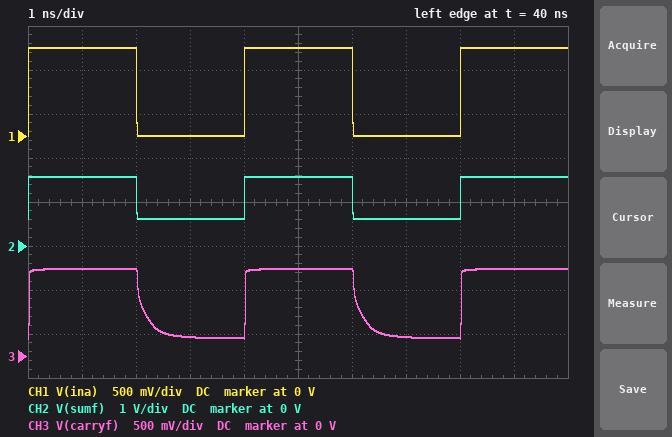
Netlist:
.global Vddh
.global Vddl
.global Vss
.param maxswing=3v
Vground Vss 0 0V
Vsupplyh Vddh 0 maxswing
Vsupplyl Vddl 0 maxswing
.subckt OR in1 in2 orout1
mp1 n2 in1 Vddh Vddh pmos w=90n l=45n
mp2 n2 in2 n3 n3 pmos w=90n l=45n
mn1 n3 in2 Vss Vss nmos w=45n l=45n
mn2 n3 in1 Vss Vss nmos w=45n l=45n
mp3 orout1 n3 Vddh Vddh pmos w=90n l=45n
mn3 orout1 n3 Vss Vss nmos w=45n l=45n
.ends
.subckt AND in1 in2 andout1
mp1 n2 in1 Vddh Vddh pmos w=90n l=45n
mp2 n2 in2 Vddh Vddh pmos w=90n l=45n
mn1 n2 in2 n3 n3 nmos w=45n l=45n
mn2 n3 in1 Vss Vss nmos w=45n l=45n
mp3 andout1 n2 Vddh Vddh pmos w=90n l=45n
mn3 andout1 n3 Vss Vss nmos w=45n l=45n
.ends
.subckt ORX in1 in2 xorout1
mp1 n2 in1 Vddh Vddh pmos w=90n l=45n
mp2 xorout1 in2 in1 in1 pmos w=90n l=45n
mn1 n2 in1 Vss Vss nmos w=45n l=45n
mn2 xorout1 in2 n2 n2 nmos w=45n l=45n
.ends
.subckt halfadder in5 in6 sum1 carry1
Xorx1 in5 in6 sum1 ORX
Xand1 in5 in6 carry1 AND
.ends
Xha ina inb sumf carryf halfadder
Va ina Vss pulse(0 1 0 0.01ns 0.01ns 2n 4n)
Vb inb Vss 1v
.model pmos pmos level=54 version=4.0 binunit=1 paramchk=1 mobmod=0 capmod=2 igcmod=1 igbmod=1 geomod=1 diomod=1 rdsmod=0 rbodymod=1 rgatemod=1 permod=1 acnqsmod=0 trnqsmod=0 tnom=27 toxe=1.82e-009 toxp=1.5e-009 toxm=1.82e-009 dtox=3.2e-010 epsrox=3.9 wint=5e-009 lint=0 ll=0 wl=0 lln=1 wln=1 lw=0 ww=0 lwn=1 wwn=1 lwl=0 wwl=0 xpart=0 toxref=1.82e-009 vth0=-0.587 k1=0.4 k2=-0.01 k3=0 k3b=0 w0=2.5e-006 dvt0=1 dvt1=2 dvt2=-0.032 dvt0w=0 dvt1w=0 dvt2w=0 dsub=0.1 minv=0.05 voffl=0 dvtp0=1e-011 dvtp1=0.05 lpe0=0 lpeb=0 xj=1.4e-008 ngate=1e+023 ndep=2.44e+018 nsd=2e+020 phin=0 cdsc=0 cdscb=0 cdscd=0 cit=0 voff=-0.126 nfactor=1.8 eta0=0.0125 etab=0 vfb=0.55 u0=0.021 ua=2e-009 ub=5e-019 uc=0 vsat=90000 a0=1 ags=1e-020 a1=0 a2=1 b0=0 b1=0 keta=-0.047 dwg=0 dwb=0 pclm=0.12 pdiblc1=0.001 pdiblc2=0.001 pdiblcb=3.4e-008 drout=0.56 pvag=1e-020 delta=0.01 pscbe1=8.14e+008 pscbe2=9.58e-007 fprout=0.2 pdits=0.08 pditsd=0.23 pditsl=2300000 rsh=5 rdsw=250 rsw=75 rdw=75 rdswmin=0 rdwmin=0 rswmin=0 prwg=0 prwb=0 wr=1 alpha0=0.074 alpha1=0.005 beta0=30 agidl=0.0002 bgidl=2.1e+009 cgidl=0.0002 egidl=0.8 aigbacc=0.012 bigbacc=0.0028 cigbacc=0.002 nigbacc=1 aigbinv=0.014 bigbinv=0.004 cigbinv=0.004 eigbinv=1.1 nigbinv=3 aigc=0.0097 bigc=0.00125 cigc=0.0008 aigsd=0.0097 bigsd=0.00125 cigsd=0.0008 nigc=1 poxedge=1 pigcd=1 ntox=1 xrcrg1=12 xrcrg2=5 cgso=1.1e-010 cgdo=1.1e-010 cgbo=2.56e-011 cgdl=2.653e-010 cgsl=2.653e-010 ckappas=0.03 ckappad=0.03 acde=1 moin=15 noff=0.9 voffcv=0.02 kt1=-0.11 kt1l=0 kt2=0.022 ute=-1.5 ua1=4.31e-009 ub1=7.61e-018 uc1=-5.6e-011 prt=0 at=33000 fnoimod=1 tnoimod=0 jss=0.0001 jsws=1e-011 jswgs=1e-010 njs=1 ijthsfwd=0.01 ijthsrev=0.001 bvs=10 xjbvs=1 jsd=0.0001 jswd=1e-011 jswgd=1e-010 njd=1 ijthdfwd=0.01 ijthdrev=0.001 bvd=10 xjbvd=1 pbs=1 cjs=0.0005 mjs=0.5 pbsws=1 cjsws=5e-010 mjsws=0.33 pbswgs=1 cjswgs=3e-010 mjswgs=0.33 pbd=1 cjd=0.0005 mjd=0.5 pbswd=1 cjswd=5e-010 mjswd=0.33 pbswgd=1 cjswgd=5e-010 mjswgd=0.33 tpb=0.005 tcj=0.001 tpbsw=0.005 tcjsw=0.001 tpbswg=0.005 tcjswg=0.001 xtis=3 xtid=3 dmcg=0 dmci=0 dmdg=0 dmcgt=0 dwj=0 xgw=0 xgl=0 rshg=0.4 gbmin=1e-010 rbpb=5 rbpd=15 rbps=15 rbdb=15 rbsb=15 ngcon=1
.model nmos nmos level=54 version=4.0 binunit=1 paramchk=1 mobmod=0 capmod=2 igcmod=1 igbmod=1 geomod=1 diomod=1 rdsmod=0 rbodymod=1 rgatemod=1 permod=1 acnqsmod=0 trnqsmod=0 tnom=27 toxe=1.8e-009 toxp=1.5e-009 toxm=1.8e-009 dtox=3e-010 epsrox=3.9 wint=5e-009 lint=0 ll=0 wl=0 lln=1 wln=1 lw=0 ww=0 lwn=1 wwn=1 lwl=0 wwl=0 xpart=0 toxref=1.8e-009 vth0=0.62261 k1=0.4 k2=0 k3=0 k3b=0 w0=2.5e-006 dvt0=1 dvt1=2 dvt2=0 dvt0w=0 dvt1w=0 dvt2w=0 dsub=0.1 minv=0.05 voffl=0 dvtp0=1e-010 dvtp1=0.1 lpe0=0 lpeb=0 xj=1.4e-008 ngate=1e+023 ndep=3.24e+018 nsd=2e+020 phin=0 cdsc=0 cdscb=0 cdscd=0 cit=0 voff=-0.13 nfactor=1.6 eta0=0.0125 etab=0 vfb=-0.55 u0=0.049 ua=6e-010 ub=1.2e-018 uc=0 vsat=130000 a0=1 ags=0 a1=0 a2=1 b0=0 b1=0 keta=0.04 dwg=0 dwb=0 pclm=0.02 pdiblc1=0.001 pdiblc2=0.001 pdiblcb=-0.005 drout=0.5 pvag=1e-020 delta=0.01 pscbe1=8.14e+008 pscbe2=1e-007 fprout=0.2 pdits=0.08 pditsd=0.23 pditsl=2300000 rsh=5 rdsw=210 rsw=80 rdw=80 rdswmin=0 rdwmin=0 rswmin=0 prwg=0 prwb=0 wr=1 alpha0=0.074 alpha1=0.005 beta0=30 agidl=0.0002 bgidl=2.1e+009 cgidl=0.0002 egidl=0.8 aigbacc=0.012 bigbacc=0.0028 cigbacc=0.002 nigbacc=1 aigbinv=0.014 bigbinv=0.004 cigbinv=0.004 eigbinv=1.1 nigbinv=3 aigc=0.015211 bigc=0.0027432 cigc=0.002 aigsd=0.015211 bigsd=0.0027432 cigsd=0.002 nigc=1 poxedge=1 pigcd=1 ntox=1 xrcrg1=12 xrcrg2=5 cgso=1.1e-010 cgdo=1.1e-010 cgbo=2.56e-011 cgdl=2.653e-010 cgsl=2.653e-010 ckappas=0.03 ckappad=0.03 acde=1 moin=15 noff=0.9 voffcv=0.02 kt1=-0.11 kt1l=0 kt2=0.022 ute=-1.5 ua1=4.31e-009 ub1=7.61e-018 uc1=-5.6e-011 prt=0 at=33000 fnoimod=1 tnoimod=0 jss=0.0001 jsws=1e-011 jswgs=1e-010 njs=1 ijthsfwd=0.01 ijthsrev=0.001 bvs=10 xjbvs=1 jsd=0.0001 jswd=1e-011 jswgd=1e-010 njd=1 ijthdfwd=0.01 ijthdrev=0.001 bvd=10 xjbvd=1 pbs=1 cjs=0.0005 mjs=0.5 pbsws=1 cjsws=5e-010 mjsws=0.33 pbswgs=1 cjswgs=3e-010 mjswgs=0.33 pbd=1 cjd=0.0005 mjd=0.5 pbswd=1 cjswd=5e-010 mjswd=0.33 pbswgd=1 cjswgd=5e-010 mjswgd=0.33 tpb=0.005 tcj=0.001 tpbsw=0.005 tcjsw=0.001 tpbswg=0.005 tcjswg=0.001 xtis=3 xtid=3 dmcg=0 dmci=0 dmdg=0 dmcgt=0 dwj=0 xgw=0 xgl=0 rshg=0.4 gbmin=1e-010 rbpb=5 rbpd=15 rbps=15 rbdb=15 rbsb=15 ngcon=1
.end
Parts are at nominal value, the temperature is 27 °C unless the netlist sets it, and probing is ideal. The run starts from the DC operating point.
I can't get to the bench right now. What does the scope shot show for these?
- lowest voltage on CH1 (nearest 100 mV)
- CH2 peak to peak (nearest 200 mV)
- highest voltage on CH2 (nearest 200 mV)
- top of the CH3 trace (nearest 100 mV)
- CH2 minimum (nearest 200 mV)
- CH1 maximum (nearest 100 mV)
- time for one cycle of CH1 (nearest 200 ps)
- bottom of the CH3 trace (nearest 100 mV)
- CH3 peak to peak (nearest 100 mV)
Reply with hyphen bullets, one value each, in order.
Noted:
- 0 V
- 1.0 V
- 1.6 V
- 1.0 V
- 600 mV
- 1.0 V
- 4.0 ns
- 200 mV
- 800 mV
